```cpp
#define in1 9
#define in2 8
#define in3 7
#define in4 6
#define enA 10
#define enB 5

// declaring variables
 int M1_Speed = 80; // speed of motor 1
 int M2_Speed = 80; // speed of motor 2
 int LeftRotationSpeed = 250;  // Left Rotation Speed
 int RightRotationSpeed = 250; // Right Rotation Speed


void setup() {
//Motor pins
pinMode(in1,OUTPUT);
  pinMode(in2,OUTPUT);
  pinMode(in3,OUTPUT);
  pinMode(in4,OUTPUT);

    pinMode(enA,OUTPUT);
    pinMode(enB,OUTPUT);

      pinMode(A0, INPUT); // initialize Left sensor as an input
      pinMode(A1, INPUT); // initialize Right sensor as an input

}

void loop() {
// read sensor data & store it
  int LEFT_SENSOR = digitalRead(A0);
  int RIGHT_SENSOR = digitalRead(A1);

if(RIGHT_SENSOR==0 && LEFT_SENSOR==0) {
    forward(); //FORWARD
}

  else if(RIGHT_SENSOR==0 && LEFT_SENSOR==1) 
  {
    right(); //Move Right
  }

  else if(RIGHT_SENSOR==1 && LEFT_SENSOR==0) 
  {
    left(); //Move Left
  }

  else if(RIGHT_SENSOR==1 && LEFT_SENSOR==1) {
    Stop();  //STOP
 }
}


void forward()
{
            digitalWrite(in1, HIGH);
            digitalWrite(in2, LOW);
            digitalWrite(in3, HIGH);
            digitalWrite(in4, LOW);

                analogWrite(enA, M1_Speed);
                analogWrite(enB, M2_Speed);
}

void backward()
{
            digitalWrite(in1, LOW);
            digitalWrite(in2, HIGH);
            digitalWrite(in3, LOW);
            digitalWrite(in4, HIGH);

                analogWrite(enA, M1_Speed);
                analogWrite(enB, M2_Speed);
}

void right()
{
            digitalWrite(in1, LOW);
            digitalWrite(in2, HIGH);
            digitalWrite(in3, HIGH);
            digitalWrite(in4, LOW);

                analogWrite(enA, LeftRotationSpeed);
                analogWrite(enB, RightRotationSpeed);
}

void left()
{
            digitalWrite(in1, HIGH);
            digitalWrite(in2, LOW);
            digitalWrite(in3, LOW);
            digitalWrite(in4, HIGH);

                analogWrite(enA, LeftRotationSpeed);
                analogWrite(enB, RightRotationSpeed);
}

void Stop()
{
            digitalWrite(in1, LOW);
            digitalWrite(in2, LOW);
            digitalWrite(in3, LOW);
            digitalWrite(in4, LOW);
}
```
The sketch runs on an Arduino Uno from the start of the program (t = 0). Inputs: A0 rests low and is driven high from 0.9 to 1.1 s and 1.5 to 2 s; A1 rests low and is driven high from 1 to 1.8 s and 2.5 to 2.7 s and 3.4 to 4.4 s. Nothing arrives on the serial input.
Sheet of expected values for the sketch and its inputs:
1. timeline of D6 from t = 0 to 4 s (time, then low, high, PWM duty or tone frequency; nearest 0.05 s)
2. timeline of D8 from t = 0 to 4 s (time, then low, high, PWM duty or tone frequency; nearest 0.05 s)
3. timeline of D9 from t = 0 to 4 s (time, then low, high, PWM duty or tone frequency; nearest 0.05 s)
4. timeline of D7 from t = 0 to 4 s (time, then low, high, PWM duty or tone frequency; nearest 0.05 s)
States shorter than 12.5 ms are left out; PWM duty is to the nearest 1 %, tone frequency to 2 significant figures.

0 s low; 1.1 s high; 1.5 s low; 2.5 s high; 2.7 s low; 3.4 s high
0 s low; 0.9 s high; 1 s low; 1.8 s high; 2 s low
0 s high; 0.9 s low; 1.1 s high; 1.5 s low; 2 s high
0 s high; 1 s low; 1.8 s high; 2.5 s low; 2.7 s high; 3.4 s low
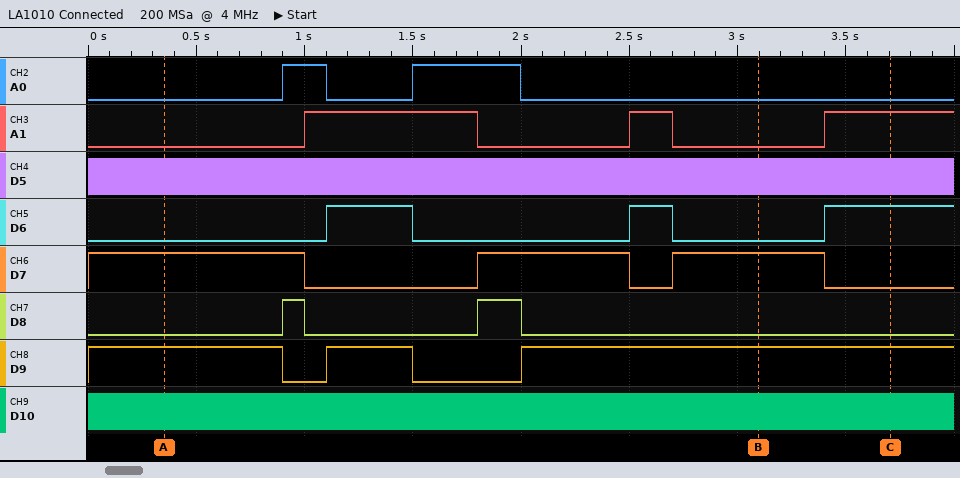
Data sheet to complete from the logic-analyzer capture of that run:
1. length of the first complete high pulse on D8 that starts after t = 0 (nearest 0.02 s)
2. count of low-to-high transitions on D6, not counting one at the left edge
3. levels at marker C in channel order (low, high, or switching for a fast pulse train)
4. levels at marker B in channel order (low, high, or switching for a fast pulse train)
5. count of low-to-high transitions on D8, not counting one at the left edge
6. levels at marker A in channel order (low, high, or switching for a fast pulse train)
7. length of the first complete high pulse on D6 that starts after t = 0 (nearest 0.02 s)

0.10 s
3
A0 low, A1 high, D5 switching, D6 high, D7 low, D8 low, D9 high, D10 switching
A0 low, A1 low, D5 switching, D6 low, D7 high, D8 low, D9 high, D10 switching
2
A0 low, A1 low, D5 switching, D6 low, D7 high, D8 low, D9 high, D10 switching
0.40 s
